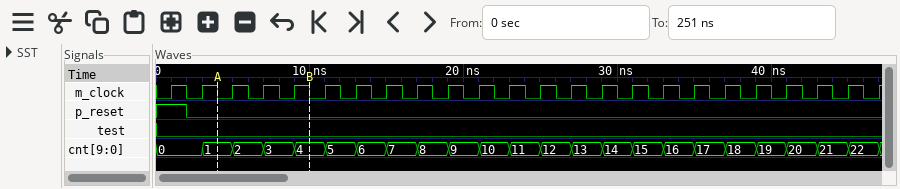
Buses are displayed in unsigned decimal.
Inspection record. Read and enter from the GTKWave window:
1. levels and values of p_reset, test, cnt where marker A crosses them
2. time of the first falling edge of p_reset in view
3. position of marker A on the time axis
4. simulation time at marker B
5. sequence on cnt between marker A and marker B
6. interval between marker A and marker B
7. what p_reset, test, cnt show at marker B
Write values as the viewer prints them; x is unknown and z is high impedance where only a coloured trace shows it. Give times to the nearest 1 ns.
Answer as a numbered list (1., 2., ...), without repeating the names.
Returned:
1. p_reset=0, test=0, cnt=1
2. 2 ns
3. 4 ns
4. 10 ns
5. 1, 2, 3, 4
6. 6 ns
7. p_reset=0, test=0, cnt=4
